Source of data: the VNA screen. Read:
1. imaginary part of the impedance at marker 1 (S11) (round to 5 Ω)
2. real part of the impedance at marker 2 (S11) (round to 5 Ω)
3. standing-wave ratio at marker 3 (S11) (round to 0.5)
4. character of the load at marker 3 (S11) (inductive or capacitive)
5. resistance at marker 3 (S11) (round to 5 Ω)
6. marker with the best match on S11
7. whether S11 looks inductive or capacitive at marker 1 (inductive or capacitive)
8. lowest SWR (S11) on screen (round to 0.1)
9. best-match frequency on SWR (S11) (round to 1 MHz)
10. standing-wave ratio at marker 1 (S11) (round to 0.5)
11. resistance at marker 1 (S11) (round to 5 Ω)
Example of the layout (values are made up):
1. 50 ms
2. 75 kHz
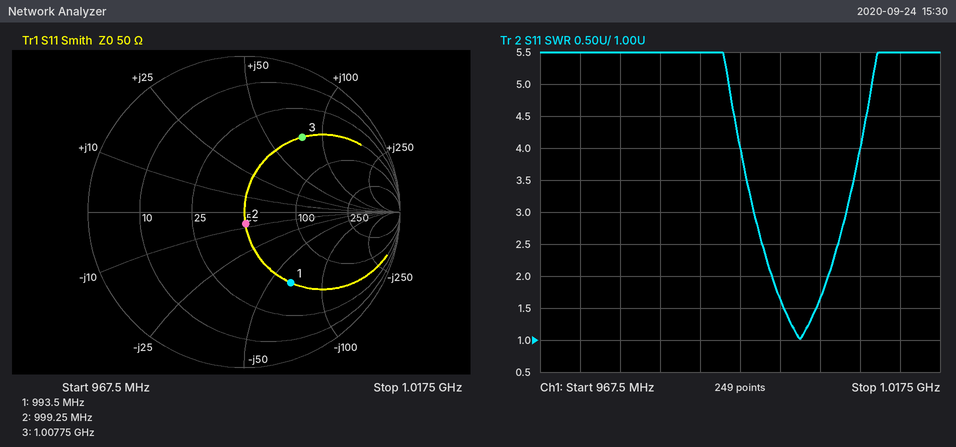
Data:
1. -65 Ω
2. 50 Ω
3. 4.0
4. inductive
5. 50 Ω
6. marker 2
7. capacitive
8. 1.0
9. 1.000 GHz
10. 3.5
11. 50 Ω
